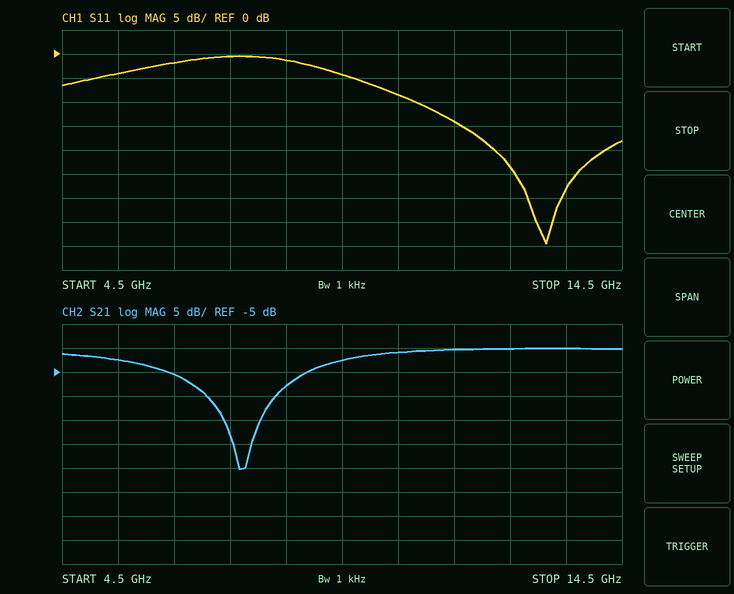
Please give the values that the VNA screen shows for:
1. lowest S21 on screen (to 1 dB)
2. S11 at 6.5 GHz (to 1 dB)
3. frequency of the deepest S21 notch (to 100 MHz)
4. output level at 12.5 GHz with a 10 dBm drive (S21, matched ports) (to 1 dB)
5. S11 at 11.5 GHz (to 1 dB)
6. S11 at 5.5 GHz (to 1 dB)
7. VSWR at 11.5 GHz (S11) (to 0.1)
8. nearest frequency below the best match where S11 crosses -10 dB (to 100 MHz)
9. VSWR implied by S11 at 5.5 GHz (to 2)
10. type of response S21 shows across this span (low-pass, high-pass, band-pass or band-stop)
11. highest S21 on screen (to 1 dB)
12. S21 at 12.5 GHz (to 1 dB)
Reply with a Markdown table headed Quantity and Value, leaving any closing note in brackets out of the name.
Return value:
| Quantity | Value |
|---|---|
| lowest S21 on screen | -25 dB |
| S11 at 6.5 GHz | -2 dB |
| frequency of the deepest S21 notch | 7.7 GHz |
| output level at 12.5 GHz with a 10 dBm drive (S21, matched ports) | 10 dBm |
| S11 at 11.5 GHz | -14 dB |
| S11 at 5.5 GHz | -4 dB |
| VSWR at 11.5 GHz (S11) | 1.5 |
| nearest frequency below the best match where S11 crosses -10 dB | 10.8 GHz |
| VSWR implied by S11 at 5.5 GHz | 4 |
| type of response S21 shows across this span | band-stop |
| highest S21 on screen | 0 dB |
| S21 at 12.5 GHz | 0 dB |
